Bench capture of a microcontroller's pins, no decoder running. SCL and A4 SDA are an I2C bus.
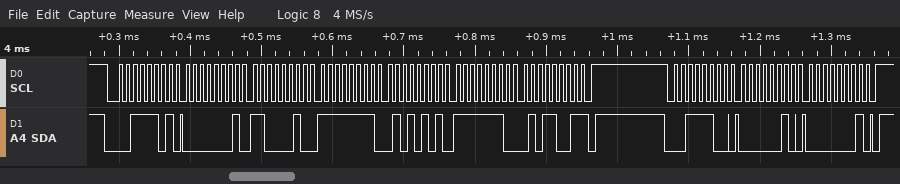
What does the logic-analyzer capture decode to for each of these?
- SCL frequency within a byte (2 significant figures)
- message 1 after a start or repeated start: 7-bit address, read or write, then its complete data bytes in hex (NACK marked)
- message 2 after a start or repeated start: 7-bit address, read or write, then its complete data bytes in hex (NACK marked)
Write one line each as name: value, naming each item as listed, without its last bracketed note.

SCL frequency within a byte: 100 kHz
message 1 after a start or repeated start: 7-bit address, read or write, then its complete data bytes in hex: 0x1E read: 01 C2 FF 55 FE 59 NACK
message 2 after a start or repeated start: 7-bit address, read or write, then its complete data bytes in hex: 0x1E write: 02 01
